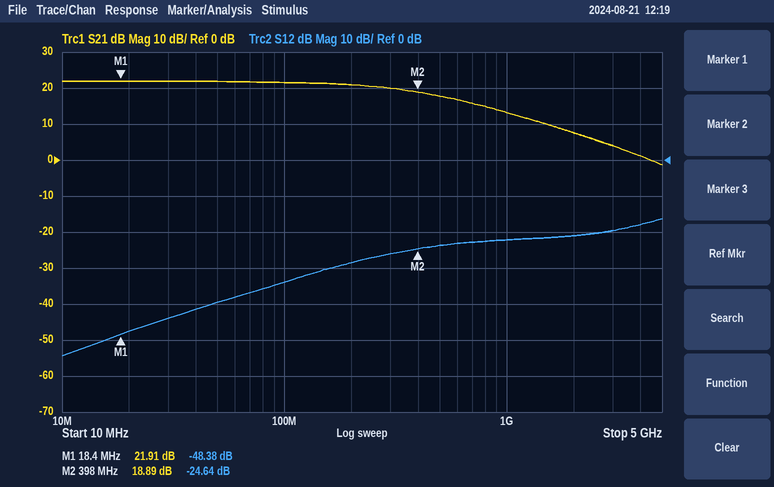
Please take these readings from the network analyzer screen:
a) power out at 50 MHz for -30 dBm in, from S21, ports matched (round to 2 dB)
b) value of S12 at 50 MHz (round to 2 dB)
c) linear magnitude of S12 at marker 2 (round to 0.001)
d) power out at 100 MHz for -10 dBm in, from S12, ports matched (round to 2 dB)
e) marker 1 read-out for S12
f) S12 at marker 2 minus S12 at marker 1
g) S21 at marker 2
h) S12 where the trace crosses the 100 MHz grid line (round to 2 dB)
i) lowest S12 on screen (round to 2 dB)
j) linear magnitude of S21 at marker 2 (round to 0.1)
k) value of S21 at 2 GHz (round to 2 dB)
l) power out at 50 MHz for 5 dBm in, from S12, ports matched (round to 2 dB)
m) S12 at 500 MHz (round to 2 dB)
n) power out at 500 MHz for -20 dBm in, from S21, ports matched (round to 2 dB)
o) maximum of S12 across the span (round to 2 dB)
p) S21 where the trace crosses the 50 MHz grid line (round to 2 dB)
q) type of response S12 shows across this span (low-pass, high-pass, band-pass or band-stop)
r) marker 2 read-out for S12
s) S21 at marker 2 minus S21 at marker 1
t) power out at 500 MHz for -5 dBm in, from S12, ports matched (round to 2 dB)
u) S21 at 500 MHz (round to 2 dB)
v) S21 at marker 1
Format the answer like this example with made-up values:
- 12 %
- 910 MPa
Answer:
- -8 dBm
- -40 dB
- 0.059
- -44 dBm
- -48.38 dB
- 23.74 dB
- 18.89 dB
- -34 dB
- -54 dB
- 8.8
- 8 dB
- -34 dBm
- -24 dB
- -2 dBm
- -16 dB
- 22 dB
- high-pass
- -24.64 dB
- -3.02 dB
- -28 dBm
- 18 dB
- 21.91 dB
